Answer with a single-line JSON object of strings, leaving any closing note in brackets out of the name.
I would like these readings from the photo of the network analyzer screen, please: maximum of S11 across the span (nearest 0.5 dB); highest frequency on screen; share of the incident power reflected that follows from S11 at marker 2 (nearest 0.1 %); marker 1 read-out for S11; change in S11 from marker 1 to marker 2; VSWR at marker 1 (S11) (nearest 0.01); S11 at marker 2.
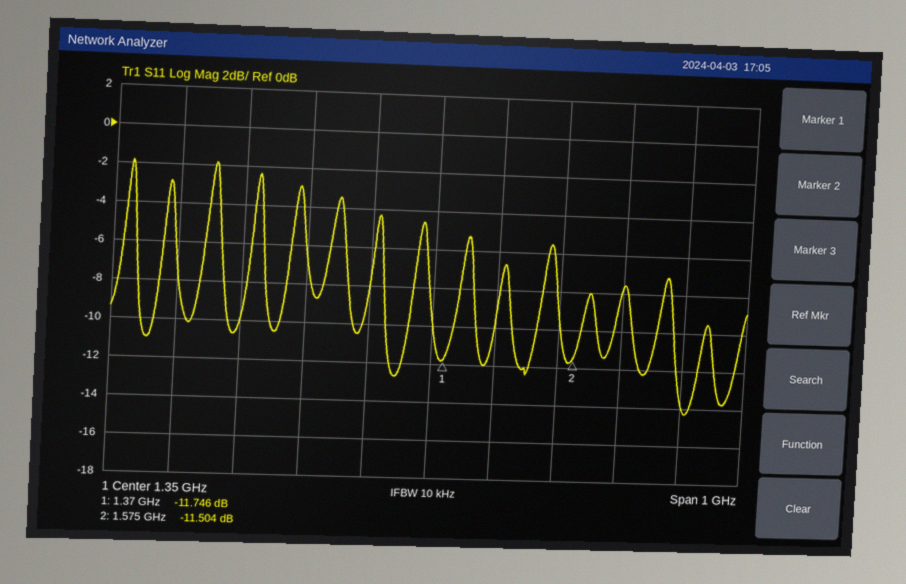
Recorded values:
{"maximum of S11 across the span": "-2.0 dB", "highest frequency on screen": "1.85 GHz", "share of the incident power reflected that follows from S11 at marker 2": "7.1 %", "marker 1 read-out for S11": "-11.746 dB", "change in S11 from marker 1 to marker 2": "0.242 dB", "VSWR at marker 1 (S11)": "1.70", "S11 at marker 2": "-11.504 dB"}
